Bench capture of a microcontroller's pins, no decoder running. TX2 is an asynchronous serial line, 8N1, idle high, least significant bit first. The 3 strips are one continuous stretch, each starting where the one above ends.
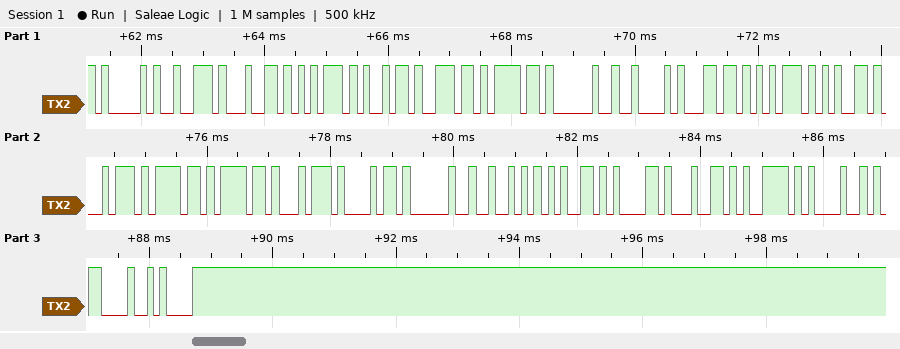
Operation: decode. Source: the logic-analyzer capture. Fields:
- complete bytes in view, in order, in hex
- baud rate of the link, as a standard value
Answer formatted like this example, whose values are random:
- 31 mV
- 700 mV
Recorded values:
- 41 72 64 75 69 6E 6F 20 42 6C 75 65 74 6F 6F 74 68 20 52 65 61 64 79 21 0D 0A
- 9600 baud
